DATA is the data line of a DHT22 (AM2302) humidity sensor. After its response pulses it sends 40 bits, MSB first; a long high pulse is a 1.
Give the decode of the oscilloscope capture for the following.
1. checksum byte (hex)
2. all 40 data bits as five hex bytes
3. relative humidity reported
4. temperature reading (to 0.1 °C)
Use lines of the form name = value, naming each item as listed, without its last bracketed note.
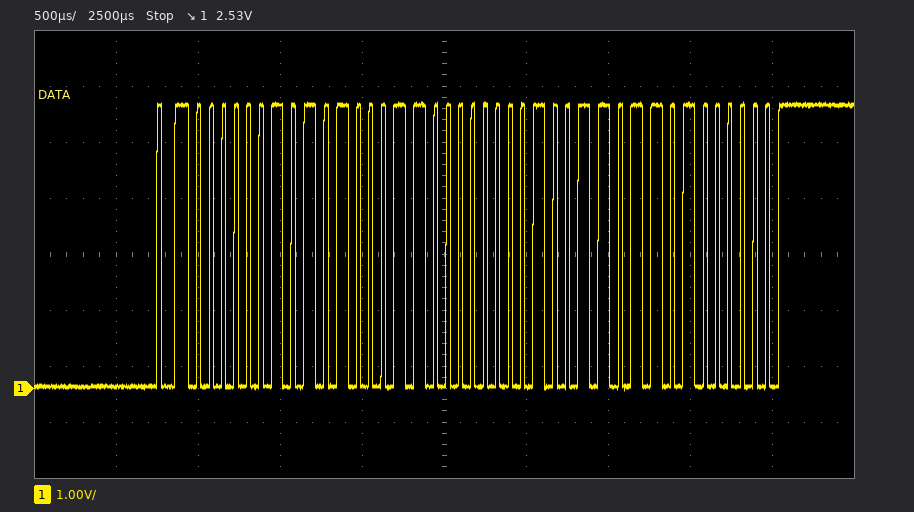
checksum byte = 0x40
all 40 data bits as five hex bytes = 02 A3 00 9B 40
relative humidity reported = 67.5 %
temperature reading = 15.5 °C
